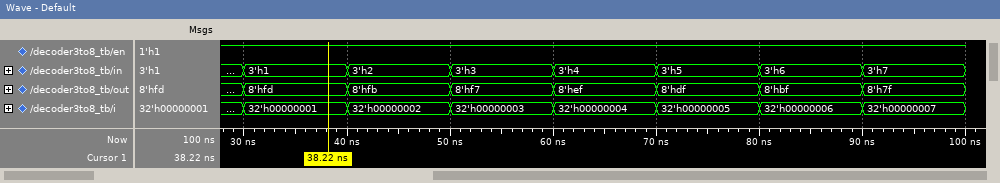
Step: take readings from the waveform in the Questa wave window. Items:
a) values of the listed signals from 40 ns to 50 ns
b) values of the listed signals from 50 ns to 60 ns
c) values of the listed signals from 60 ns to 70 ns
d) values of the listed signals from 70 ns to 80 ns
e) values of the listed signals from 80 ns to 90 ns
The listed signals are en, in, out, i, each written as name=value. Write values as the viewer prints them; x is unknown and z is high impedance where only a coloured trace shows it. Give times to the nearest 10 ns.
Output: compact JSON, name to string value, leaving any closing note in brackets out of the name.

{"values of the listed signals from 40 ns to 50 ns": "en=1, in=3'h2, out=8'hfb, i=32'h00000002", "values of the listed signals from 50 ns to 60 ns": "en=1, in=3'h3, out=8'hf7, i=32'h00000003", "values of the listed signals from 60 ns to 70 ns": "en=1, in=3'h4, out=8'hef, i=32'h00000004", "values of the listed signals from 70 ns to 80 ns": "en=1, in=3'h5, out=8'hdf, i=32'h00000005", "values of the listed signals from 80 ns to 90 ns": "en=1, in=3'h6, out=8'hbf, i=32'h00000006"}
